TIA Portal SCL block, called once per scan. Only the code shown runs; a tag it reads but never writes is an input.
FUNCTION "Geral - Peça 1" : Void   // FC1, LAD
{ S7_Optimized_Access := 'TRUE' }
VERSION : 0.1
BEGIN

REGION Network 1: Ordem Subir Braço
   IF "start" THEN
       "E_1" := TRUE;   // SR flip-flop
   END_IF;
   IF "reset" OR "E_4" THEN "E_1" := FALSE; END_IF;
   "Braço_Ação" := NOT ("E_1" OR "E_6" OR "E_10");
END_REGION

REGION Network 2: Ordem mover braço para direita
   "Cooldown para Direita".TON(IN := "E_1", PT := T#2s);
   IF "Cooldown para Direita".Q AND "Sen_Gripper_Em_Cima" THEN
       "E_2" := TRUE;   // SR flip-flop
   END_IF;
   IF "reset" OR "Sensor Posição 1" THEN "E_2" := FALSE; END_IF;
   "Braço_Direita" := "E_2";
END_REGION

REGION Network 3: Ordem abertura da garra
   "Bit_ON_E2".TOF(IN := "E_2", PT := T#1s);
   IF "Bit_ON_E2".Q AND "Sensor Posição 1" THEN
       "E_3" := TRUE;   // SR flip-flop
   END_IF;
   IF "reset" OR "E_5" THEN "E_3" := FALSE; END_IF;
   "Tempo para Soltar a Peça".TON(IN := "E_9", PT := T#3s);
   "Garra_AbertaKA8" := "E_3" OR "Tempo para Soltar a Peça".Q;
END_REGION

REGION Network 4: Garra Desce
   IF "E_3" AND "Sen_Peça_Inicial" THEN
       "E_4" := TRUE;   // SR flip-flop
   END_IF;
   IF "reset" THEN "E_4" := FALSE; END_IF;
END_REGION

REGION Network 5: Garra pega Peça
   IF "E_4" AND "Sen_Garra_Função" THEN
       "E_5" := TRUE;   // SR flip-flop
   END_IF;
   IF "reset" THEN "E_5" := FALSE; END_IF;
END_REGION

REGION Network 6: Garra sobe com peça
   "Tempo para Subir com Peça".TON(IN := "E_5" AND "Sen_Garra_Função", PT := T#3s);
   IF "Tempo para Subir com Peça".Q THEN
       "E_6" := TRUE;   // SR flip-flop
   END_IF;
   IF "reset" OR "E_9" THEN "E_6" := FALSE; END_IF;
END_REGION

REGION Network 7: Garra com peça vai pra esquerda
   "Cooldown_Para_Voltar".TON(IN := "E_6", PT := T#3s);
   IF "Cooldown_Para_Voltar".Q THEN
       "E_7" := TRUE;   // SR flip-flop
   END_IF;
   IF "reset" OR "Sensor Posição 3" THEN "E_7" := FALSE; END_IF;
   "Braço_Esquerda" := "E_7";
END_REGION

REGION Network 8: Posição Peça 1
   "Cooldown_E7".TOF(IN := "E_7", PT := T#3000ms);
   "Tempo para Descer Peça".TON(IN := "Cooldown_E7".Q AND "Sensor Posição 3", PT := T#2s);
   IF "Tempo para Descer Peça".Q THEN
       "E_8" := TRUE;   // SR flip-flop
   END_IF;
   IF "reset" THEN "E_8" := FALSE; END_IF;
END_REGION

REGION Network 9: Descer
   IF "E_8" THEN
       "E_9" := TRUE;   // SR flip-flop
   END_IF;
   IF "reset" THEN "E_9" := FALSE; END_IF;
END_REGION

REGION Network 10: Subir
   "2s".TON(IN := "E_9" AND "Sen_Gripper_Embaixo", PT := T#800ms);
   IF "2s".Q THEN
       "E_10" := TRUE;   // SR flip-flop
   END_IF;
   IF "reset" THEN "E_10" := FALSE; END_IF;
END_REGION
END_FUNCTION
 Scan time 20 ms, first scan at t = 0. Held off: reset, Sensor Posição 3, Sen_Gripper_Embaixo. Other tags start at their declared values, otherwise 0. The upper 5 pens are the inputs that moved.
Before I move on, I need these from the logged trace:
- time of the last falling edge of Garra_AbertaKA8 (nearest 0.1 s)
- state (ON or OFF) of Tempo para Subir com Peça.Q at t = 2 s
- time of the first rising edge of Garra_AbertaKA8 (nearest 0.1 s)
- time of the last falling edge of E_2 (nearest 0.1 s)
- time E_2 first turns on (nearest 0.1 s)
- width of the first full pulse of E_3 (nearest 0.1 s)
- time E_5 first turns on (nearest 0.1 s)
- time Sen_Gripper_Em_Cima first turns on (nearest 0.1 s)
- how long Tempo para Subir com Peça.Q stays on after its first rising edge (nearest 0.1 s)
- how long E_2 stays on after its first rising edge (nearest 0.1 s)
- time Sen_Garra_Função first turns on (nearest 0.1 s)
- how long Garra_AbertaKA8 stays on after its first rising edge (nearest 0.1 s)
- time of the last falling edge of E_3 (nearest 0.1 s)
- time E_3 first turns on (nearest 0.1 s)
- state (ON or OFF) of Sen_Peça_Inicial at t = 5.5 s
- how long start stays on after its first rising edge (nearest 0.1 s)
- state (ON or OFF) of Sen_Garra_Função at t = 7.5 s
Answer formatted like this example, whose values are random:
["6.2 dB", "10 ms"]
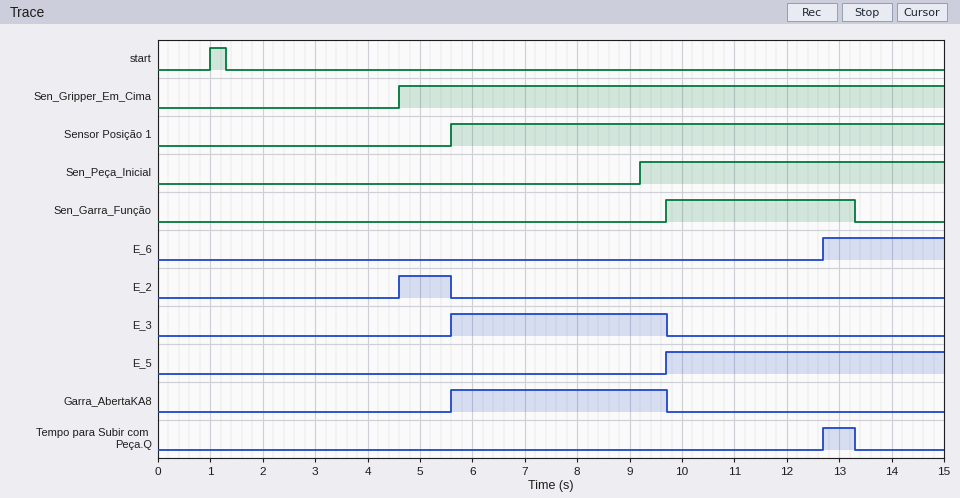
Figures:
["9.7 s", "OFF", "5.6 s", "5.6 s", "4.6 s", "4.1 s", "9.7 s", "4.6 s", "0.6 s", "1.0 s", "9.7 s", "4.1 s", "9.7 s", "5.6 s", "OFF", "0.3 s", "OFF"]
